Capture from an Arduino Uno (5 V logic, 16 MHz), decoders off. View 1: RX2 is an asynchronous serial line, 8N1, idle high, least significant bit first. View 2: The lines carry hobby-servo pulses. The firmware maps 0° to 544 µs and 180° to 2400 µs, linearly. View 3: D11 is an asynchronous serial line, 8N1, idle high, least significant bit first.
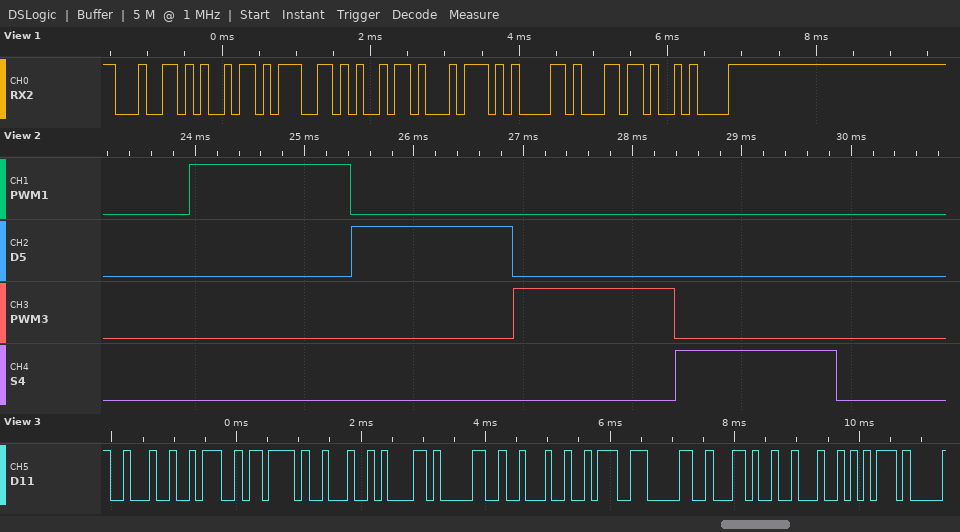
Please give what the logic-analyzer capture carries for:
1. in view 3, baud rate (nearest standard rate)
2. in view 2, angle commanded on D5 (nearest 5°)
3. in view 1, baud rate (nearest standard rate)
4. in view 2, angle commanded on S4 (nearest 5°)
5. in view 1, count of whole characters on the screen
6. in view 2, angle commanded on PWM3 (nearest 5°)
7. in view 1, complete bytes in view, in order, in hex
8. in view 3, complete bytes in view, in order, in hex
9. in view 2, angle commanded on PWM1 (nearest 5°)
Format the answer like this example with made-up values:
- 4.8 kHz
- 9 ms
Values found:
- 9600 baud
- 90°
- 9600 baud
- 90°
- 8
- 90°
- 64 69 67 69 74 61 6C 0A
- 0x22 0x3A 0x7B 0x22 0x61 0x30 0x22 0x3A 0x30 0x2C 0x22 0x75
- 90°
